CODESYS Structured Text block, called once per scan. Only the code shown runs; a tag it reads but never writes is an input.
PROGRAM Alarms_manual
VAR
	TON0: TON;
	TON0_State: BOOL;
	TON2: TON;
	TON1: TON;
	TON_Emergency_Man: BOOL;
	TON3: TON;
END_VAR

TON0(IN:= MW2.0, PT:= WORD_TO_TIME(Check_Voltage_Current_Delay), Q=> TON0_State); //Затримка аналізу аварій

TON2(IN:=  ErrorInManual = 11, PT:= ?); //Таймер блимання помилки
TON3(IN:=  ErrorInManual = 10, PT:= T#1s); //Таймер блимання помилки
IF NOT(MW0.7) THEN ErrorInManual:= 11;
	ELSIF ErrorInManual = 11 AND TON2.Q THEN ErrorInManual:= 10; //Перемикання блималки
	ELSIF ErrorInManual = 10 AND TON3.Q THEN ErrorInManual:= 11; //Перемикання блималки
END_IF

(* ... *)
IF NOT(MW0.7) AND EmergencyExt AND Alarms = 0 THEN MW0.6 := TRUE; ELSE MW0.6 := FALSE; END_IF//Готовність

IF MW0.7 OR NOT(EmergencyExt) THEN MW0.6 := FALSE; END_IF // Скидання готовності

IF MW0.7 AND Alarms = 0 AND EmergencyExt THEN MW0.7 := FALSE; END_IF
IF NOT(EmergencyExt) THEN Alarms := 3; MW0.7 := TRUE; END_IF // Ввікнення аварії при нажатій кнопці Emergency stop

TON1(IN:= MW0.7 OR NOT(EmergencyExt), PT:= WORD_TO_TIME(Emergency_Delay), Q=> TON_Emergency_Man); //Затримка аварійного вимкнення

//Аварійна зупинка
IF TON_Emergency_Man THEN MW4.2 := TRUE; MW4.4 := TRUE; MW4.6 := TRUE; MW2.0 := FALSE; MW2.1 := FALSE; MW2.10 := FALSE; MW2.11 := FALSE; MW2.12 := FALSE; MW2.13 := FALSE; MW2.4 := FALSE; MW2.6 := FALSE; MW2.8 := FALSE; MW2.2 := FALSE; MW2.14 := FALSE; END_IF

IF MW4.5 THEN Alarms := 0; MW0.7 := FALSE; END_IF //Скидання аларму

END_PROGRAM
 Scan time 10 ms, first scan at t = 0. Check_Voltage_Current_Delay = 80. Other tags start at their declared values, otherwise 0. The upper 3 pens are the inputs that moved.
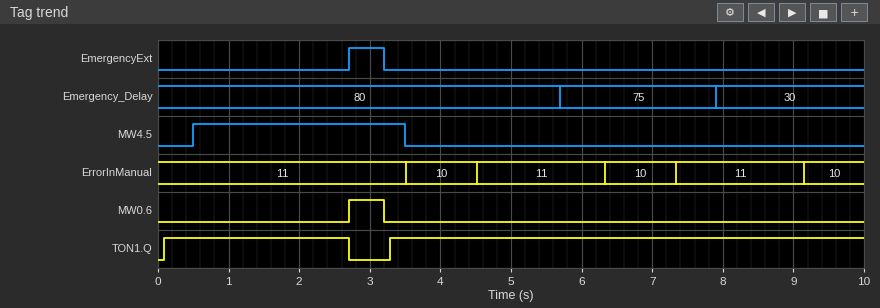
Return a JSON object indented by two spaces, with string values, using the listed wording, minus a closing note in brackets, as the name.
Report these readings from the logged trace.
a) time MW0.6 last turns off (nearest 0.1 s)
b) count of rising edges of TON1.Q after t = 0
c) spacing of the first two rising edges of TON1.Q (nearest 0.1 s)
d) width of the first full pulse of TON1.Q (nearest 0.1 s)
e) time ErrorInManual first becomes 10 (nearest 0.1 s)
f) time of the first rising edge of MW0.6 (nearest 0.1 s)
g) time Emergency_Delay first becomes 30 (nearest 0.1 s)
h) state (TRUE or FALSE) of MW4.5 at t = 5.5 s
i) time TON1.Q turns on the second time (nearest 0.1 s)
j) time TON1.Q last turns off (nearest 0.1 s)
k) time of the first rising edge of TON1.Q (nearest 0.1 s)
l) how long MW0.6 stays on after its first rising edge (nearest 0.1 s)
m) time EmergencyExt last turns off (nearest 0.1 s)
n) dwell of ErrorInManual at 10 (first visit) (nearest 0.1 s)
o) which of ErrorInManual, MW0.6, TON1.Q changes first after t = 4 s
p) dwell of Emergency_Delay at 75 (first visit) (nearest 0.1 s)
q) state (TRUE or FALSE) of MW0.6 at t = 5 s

{
  "time MW0.6 last turns off": "3.2 s",
  "count of rising edges of TON1.Q after t = 0": "2",
  "spacing of the first two rising edges of TON1.Q": "3.2 s",
  "width of the first full pulse of TON1.Q": "2.6 s",
  "time ErrorInManual first becomes 10": "3.5 s",
  "time of the first rising edge of MW0.6": "2.7 s",
  "time Emergency_Delay first becomes 30": "7.9 s",
  "state (TRUE or FALSE) of MW4.5 at t = 5.5 s": "FALSE",
  "time TON1.Q turns on the second time": "3.3 s",
  "time TON1.Q last turns off": "2.7 s",
  "time of the first rising edge of TON1.Q": "0.1 s",
  "how long MW0.6 stays on after its first rising edge": "0.5 s",
  "time EmergencyExt last turns off": "3.2 s",
  "dwell of ErrorInManual at 10 (first visit)": "1.0 s",
  "which of ErrorInManual, MW0.6, TON1.Q changes first after t = 4 s": "ErrorInManual",
  "dwell of Emergency_Delay at 75 (first visit)": "2.2 s",
  "state (TRUE or FALSE) of MW0.6 at t = 5 s": "FALSE"
}
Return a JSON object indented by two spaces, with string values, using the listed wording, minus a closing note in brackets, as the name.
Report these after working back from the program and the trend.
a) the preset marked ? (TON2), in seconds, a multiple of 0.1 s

{
  "the preset marked ? (TON2), in seconds, a multiple of 0.1 s": "1.8 s"
}
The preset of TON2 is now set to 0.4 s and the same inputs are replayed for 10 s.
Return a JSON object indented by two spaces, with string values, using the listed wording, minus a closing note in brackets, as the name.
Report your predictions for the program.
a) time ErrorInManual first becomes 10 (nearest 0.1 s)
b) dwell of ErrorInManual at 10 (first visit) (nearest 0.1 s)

{
  "time ErrorInManual first becomes 10": "0.4 s",
  "dwell of ErrorInManual at 10 (first visit)": "0.1 s"
}
